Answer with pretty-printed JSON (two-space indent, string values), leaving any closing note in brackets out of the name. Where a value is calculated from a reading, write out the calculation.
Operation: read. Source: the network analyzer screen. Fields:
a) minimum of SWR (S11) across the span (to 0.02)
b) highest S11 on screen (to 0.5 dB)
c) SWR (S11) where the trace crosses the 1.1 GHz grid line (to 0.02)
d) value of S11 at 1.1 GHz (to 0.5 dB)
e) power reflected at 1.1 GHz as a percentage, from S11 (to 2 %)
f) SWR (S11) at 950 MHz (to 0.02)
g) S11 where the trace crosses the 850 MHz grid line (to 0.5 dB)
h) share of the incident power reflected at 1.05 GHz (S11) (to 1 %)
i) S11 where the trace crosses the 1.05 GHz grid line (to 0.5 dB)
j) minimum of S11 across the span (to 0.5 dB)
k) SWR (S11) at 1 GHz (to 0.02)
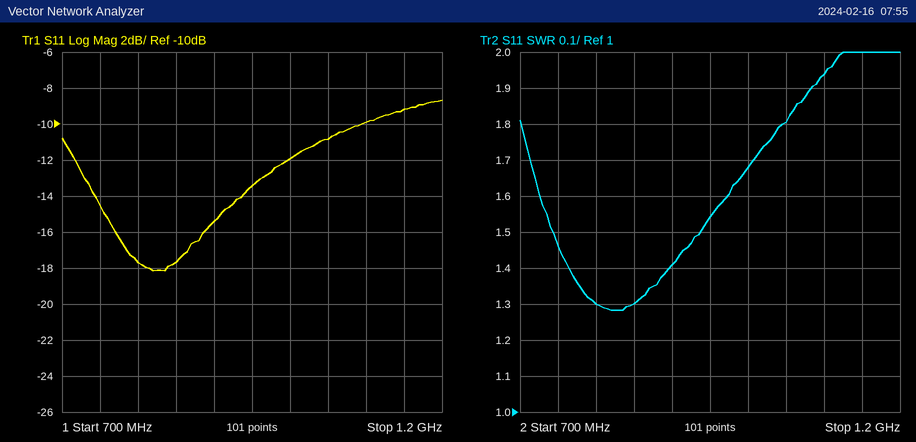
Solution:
{
  "minimum of SWR (S11) across the span": "1.28",
  "highest S11 on screen": "-8.5 dB",
  "SWR (S11) where the trace crosses the 1.1 GHz grid line": "1.94",
  "value of S11 at 1.1 GHz": "-10.0 dB",
  "power reflected at 1.1 GHz as a percentage, from S11": "10^(-10/10) ≈ 10 %",
  "SWR (S11) at 950 MHz": "1.54",
  "S11 where the trace crosses the 850 MHz grid line": "-17.5 dB",
  "share of the incident power reflected at 1.05 GHz (S11)": "10^(-11/10) ≈ 8 %",
  "S11 where the trace crosses the 1.05 GHz grid line": "-11.0 dB",
  "minimum of S11 across the span": "-18.0 dB",
  "SWR (S11) at 1 GHz": "1.68"
}
